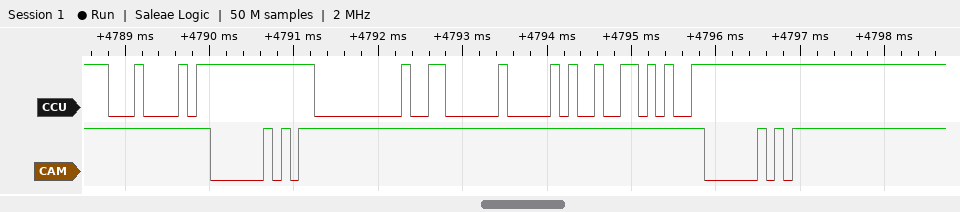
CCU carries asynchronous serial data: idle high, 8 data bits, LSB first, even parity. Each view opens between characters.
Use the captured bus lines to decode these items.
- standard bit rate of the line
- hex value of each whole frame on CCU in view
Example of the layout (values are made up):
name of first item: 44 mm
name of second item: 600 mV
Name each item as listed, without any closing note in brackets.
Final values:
standard bit rate of the line: 9600 baud
hex value of each whole frame on CCU in view: 84, 00, 06, 50, 56
